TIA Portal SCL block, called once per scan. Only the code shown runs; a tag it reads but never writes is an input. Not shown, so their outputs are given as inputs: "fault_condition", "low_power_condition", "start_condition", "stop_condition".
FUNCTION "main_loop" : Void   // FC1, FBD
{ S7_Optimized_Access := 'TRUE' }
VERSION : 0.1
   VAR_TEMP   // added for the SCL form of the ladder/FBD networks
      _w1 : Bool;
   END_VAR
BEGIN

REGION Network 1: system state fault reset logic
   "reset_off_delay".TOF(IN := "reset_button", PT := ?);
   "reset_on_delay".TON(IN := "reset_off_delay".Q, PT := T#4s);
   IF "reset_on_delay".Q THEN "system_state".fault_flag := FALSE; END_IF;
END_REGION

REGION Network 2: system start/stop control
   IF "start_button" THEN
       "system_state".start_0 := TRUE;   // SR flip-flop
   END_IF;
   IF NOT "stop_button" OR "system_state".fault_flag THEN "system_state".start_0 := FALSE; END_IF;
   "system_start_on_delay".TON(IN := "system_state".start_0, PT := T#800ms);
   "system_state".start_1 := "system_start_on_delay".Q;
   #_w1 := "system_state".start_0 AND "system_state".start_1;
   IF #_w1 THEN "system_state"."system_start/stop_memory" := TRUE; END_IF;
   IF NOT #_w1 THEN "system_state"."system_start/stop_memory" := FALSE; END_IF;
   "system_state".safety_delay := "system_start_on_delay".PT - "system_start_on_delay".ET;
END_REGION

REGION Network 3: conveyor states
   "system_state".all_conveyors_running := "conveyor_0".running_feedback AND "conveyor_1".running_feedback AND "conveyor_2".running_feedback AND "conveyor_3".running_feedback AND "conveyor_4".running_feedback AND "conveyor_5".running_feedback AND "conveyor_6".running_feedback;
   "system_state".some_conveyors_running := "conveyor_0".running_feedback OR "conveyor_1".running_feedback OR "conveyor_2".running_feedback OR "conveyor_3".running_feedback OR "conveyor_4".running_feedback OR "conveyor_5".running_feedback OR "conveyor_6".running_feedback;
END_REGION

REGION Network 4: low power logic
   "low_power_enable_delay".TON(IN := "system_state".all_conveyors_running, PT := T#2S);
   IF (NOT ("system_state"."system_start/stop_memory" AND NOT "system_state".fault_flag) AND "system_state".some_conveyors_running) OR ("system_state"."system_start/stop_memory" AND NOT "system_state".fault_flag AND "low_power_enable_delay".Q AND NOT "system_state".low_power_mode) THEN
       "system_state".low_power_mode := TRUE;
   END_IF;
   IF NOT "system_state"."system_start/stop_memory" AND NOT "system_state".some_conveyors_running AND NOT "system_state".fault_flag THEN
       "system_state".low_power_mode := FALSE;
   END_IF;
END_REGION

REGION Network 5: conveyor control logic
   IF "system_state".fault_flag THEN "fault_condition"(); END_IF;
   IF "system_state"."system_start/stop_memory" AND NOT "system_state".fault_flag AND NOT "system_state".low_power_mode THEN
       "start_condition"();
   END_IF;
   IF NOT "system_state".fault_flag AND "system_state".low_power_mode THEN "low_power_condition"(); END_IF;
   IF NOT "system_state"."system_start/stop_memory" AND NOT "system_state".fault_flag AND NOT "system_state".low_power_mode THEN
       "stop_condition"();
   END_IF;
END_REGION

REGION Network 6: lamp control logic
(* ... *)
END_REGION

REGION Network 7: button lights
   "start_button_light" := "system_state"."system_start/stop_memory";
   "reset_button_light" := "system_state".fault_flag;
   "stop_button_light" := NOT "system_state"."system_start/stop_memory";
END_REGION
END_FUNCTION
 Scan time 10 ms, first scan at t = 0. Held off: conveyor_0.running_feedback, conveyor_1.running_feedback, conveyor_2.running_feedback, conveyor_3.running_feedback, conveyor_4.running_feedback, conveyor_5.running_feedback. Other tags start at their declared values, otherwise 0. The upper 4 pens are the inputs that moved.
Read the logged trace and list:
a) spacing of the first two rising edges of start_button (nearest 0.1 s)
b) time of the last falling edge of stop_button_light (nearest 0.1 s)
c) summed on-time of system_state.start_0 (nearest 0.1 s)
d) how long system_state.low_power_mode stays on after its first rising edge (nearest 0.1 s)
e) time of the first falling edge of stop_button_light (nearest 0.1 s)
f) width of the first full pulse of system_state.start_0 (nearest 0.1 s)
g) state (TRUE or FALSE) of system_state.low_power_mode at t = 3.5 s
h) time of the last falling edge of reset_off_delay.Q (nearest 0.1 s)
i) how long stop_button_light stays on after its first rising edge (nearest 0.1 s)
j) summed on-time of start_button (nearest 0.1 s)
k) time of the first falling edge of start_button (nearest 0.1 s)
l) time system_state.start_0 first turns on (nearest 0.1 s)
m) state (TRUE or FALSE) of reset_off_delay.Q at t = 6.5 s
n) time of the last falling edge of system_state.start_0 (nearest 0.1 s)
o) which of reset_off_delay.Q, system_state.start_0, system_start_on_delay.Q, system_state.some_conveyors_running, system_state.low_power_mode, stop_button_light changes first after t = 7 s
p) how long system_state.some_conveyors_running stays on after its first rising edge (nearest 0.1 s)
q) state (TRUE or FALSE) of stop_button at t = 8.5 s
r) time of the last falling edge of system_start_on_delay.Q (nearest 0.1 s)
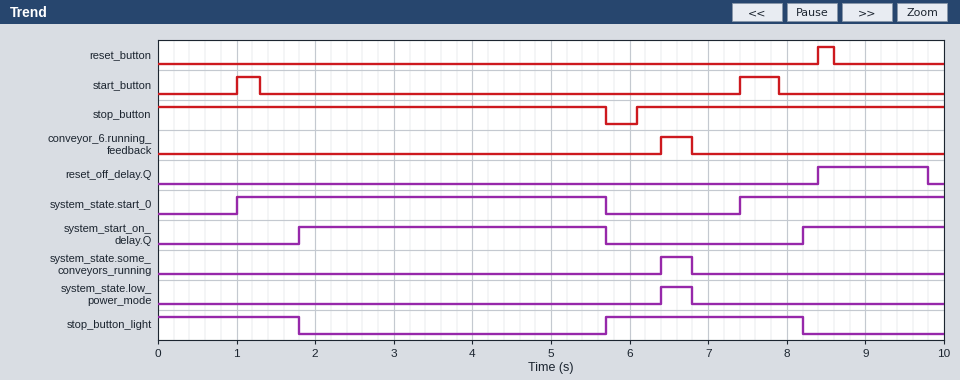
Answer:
6.4 s
8.2 s
7.3 s
0.4 s
1.8 s
4.7 s
FALSE
9.8 s
2.5 s
0.8 s
1.3 s
1.0 s
FALSE
5.7 s
system_state.start_0
0.4 s
TRUE
5.7 s
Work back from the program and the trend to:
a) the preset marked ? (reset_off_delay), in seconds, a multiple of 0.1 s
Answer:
1.2 s
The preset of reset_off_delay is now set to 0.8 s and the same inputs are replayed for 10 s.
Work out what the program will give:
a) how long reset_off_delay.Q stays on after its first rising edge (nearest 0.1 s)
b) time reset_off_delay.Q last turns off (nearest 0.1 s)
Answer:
1.0 s
9.4 s
